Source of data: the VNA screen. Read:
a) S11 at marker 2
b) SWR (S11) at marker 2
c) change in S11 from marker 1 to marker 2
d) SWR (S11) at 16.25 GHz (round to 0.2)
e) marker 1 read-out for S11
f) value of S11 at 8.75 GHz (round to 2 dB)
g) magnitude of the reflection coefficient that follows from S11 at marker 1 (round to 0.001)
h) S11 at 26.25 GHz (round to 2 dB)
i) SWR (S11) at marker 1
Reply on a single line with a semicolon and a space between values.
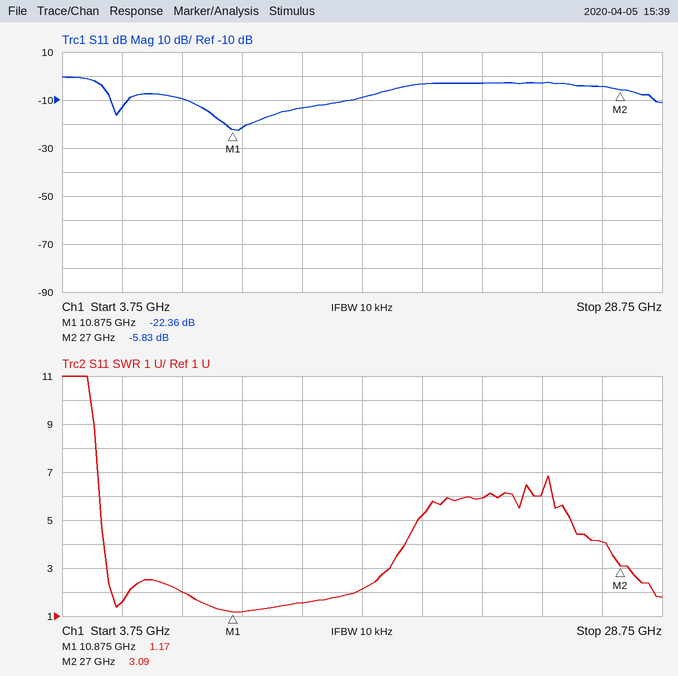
-5.83 dB; 3.09; 16.53 dB; 2.2; -22.36 dB; -10 dB; 0.076; -4 dB; 1.17
